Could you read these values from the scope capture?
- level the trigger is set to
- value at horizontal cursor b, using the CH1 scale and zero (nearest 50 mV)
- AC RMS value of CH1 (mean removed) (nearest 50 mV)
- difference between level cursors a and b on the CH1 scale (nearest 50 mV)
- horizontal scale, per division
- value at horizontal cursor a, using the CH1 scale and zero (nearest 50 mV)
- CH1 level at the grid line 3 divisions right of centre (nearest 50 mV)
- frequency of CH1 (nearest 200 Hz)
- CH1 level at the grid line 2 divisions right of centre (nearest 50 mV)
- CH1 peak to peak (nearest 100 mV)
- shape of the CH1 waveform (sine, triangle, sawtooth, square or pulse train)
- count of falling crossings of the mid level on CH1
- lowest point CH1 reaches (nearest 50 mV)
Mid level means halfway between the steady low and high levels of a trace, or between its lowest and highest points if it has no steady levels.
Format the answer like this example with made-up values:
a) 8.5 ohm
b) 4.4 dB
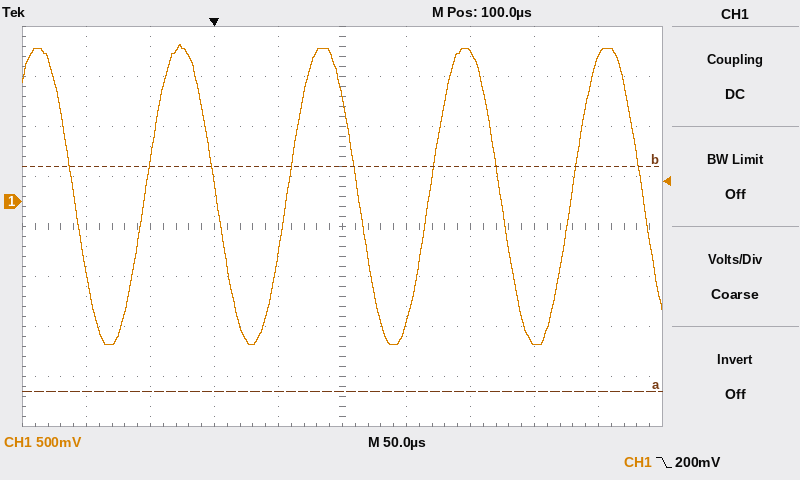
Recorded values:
a) 200 mV
b) 350 mV
c) 1.05 V
d) 2.25 V
e) 50 µs
f) -1.90 V
g) -1.40 V
h) 9.0 kHz
i) 1.50 V
j) 3.00 V
k) sine
l) 5
m) -1.45 V
